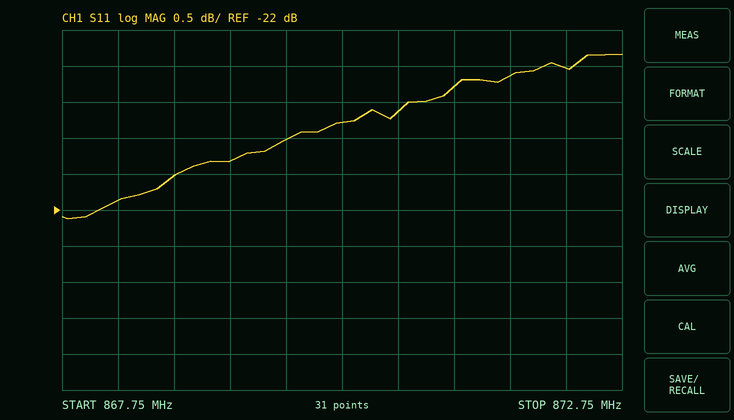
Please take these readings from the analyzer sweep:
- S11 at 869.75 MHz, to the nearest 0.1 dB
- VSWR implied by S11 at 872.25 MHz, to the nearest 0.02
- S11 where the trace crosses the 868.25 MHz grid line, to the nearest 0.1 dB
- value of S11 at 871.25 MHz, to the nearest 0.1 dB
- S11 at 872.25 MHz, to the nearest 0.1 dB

-21.0 dB
1.22
-21.9 dB
-20.3 dB
-20.0 dB
